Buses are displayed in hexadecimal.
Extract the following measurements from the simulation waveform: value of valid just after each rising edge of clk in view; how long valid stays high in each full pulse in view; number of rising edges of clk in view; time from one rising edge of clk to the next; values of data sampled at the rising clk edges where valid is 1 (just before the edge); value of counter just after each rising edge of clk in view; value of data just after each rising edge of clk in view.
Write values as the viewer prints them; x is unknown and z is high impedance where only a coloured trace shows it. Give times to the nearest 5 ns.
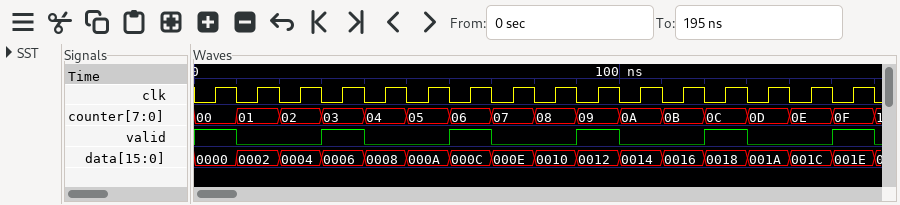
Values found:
1 0 0 1 0 0 1 0 0 1 0 0 1 0 0 1
10 ns, 10 ns, 10 ns, 10 ns, 10 ns
16
10 ns
0000, 0006, 000C, 0012, 0018, 001E
00, 01, 02, 03, 04, 05, 06, 07, 08, 09, 0A, 0B, 0C, 0D, 0E, 0F
0000, 0002, 0004, 0006, 0008, 000A, 000C, 000E, 0010, 0012, 0014, 0016, 0018, 001A, 001C, 001E
